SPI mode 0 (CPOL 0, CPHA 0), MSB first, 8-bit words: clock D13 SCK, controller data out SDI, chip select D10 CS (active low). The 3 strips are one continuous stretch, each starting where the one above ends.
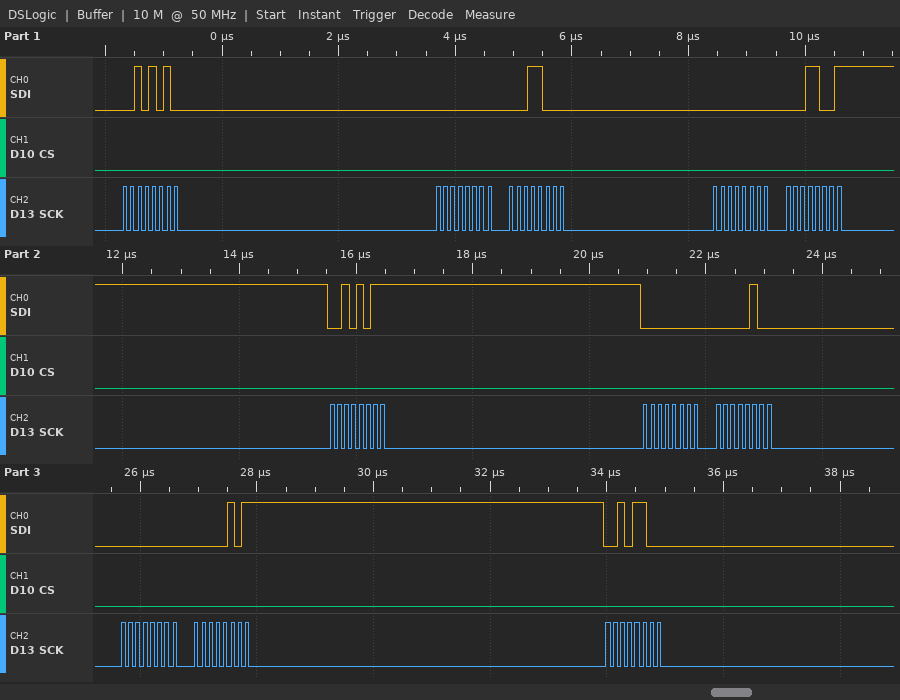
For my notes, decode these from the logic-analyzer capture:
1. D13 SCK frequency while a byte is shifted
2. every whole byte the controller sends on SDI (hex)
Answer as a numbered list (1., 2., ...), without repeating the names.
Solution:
1. 8 MHz
2. 2A 00 18 00 19 2B 00 04 00 05 2C
